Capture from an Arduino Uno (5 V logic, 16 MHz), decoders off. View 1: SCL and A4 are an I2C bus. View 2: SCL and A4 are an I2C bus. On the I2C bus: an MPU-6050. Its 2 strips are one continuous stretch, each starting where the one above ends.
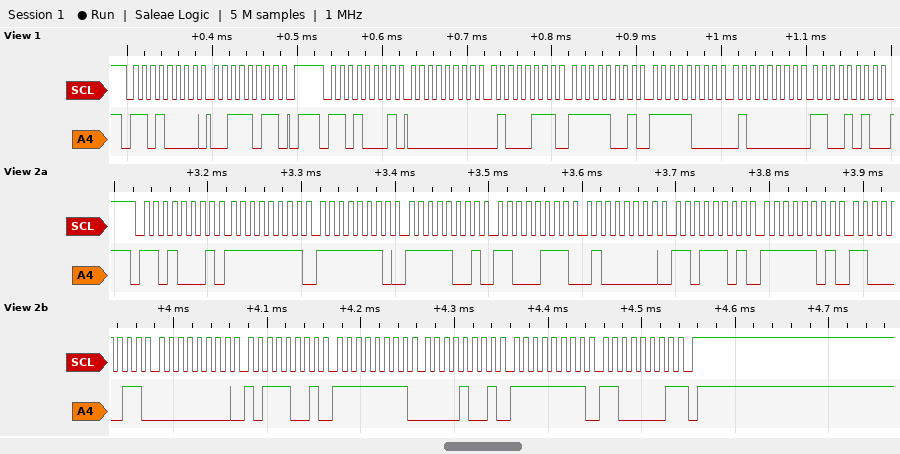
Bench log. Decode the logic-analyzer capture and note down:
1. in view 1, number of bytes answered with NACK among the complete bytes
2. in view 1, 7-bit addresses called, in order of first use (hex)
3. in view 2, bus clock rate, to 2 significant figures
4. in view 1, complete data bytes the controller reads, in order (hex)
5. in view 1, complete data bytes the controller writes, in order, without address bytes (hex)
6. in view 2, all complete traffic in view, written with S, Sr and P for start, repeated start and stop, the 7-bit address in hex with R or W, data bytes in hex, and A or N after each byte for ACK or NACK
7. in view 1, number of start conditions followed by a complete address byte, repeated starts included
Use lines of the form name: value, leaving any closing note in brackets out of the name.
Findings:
in view 1, number of bytes answered with NACK among the complete bytes: 0
in view 1, 7-bit addresses called, in order of first use: 0x68
in view 2, bus clock rate, to 2 significant figures: 100 kHz
in view 1, complete data bytes the controller reads, in order: 00 47 F9 F8 40 CA
in view 1, complete data bytes the controller writes, in order, without address bytes: 3B
in view 2, all complete traffic in view, written with S, Sr and P for start, repeated start and stop, the 7-bit address in hex with R or W, data bytes in hex, and A or N after each byte for ACK or NACK: S 68R A FF A FE A F9 A C7 A 40 A DD A FD A C3 A 00 A B9 A FF A 09 A FF A C1 N P
in view 1, number of start conditions followed by a complete address byte, repeated starts included: 2
